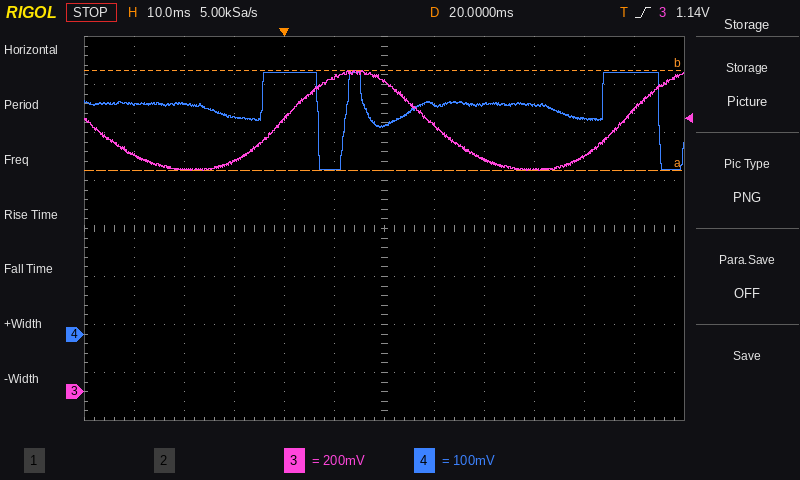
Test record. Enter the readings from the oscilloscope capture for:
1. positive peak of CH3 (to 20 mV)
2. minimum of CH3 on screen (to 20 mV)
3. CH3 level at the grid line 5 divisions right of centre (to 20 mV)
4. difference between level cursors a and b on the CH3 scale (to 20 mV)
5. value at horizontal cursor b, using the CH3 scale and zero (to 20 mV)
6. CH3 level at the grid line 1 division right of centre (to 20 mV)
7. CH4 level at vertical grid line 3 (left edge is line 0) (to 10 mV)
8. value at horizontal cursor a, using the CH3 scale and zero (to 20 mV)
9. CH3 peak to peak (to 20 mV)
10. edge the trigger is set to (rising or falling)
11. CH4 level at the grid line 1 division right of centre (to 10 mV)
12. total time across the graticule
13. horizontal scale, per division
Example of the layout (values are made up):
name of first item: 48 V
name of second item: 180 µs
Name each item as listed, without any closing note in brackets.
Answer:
positive peak of CH3: 1.34 V
minimum of CH3 on screen: 920 mV
CH3 level at the grid line 5 divisions right of centre: 1.18 V
difference between level cursors a and b on the CH3 scale: 420 mV
value at horizontal cursor b, using the CH3 scale and zero: 1.34 V
CH3 level at the grid line 1 division right of centre: 1.10 V
CH4 level at vertical grid line 3 (left edge is line 0): 450 mV
value at horizontal cursor a, using the CH3 scale and zero: 920 mV
CH3 peak to peak: 420 mV
edge the trigger is set to: rising
CH4 level at the grid line 1 division right of centre: 480 mV
total time across the graticule: 120 ms
horizontal scale, per division: 10 ms
